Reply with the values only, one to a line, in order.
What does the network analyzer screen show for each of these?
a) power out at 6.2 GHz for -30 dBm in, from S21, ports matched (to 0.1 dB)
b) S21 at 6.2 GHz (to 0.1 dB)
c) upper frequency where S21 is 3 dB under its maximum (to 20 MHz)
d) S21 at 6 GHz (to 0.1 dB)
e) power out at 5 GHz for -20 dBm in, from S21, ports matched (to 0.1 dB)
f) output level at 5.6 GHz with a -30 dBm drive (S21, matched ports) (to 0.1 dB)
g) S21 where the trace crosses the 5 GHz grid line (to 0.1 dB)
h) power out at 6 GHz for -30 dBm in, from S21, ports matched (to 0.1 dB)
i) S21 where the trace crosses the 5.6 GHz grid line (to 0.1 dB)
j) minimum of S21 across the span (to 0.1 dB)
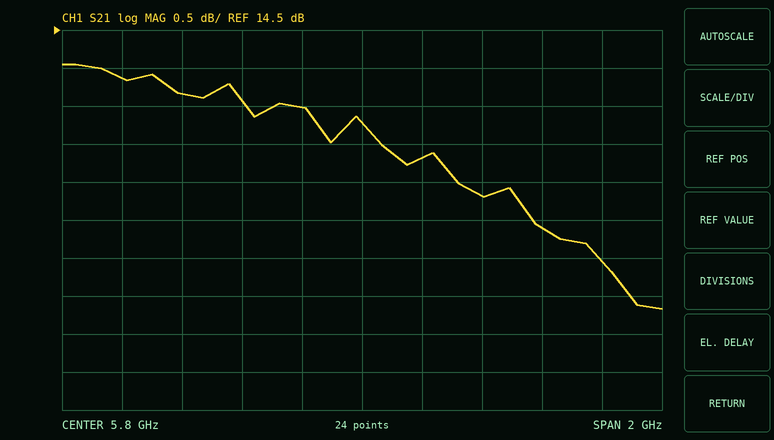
-17.7 dBm
12.3 dB
6.68 GHz
12.8 dB
-6.1 dBm
-16.5 dBm
13.9 dB
-17.2 dBm
13.5 dB
10.8 dB
